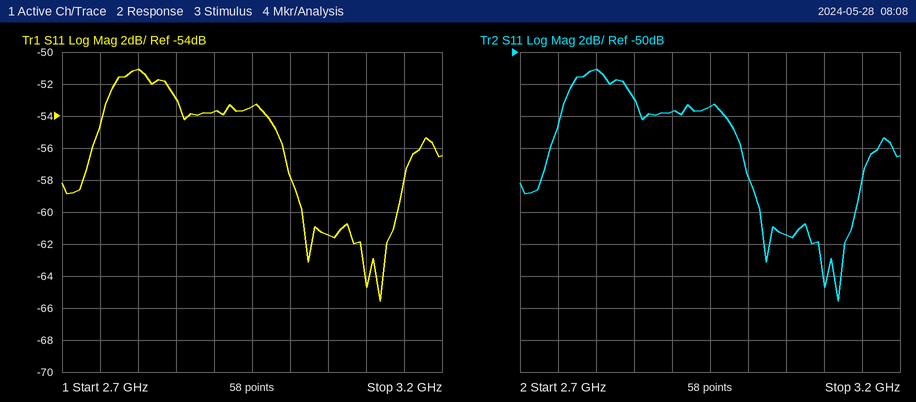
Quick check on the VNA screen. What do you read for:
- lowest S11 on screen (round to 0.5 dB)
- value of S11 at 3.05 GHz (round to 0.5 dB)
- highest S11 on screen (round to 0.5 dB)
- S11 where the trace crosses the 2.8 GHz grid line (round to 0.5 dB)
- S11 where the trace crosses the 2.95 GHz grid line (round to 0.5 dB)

-65.5 dB
-61.5 dB
-51.0 dB
-51.0 dB
-53.5 dB
